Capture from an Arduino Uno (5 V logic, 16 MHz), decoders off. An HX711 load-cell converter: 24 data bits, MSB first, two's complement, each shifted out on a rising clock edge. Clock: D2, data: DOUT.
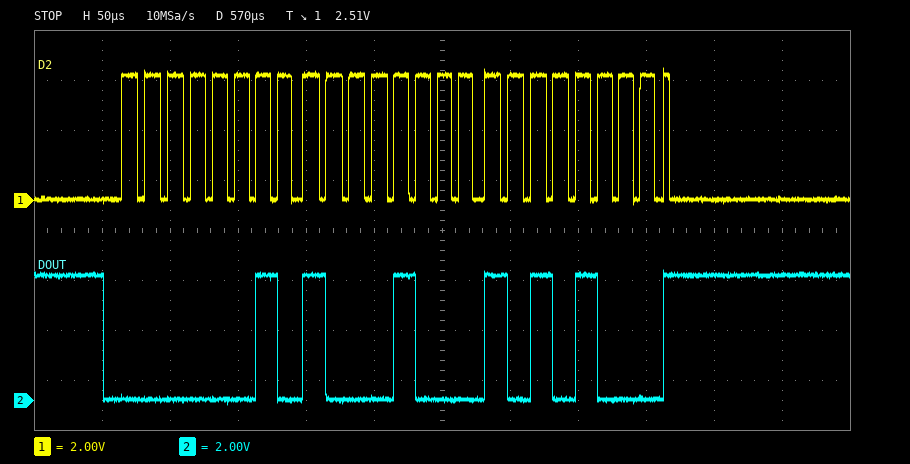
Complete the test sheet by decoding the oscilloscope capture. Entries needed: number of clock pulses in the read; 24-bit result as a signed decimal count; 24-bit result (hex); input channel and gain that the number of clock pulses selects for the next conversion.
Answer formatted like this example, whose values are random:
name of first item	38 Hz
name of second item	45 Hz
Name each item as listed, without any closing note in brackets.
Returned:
number of clock pulses in the read	25
24-bit result as a signed decimal count	166056
24-bit result	0x0288A8
input channel and gain that the number of clock pulses selects for the next conversion	channel A, gain 128
